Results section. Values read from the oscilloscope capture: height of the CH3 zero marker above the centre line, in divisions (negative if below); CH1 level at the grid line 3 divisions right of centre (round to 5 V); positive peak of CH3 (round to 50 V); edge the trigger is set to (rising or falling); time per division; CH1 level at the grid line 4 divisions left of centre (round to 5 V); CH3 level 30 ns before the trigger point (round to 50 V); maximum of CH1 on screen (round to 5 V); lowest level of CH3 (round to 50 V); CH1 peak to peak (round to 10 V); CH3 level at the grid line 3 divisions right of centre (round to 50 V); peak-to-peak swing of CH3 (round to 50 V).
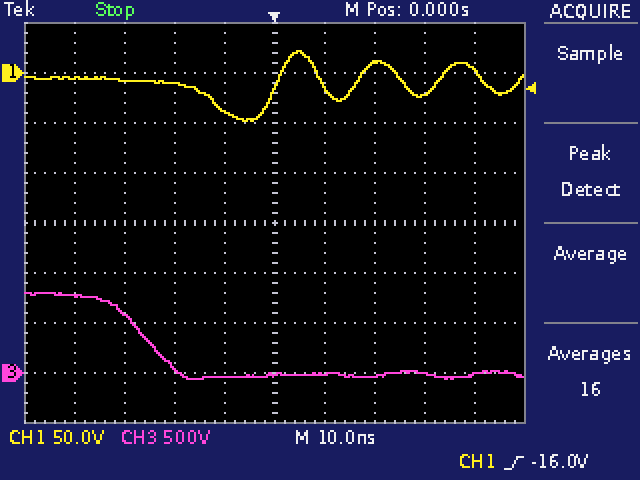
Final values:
-3.0 div
-20 V
800 V
rising
10 ns
-5 V
600 V
20 V
-50 V
70 V
0 V
850 V
